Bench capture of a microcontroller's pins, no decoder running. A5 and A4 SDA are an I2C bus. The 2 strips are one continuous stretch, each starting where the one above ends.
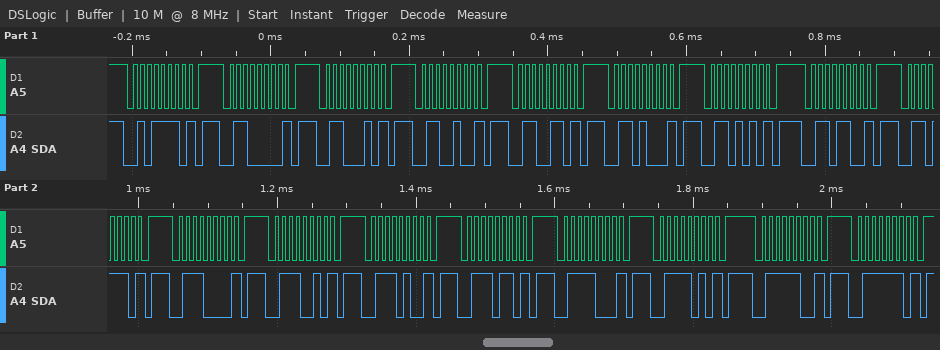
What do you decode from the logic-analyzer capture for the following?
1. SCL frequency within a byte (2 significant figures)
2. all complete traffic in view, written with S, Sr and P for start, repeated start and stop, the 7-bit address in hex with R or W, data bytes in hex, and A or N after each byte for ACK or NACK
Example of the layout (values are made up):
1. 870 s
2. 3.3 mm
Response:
1. 100 kHz
2. S 2FW N P S 30W N P S 31W N P S 32W N P S 33W N P S 34W N P S 35W N P S 36W N P S 37W N P S 38W N P S 39W N P S 3AW N P S 3BW N P S 3CW N P S 3DW N P S 3EW N P S 3FW N P
